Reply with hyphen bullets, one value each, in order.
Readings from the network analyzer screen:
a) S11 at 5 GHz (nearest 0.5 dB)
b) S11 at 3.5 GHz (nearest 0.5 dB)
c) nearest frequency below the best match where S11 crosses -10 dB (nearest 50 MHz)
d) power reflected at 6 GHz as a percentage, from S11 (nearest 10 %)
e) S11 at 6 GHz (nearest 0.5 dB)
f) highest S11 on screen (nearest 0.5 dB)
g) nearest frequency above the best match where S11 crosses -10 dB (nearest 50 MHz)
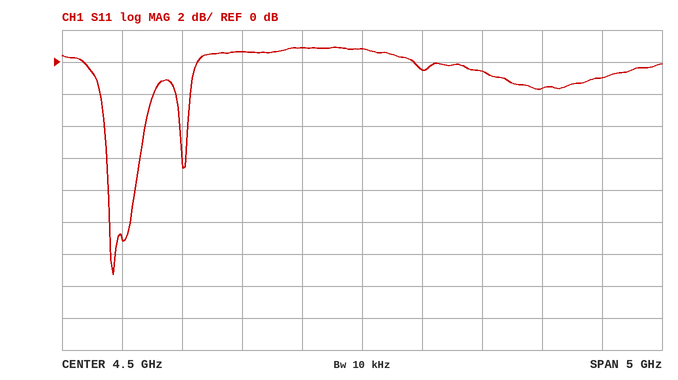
- -0.5 dB
- 0.5 dB
- 2.40 GHz
- 70 %
- -1.5 dB
- 1.0 dB
- 2.55 GHz
